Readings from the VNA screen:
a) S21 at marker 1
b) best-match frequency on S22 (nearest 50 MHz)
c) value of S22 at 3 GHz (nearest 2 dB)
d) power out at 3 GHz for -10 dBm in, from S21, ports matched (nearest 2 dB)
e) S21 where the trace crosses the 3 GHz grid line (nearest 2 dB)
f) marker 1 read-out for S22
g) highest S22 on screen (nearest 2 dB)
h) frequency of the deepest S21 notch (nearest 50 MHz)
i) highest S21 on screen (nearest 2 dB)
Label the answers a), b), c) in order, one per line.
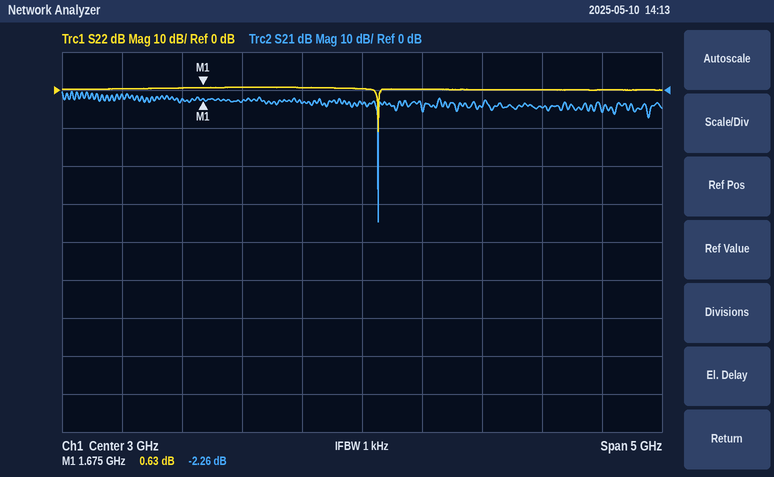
a) -2.26 dB
b) 3.15 GHz
c) 0 dB
d) -14 dBm
e) -4 dB
f) 0.63 dB
g) 0 dB
h) 3.15 GHz
i) 0 dB
